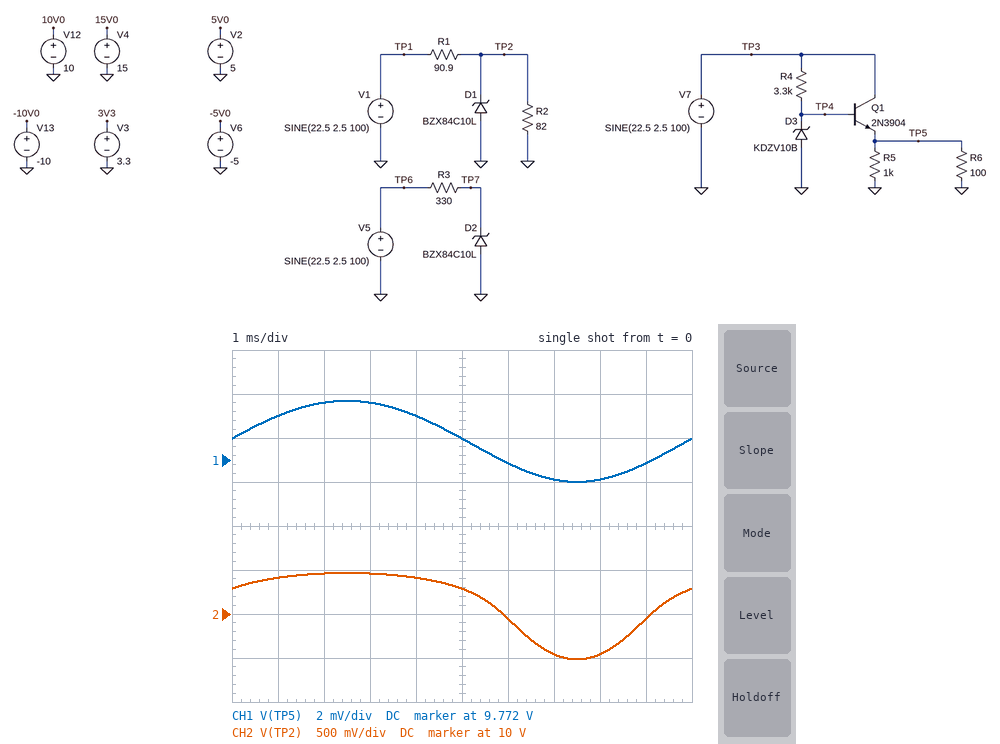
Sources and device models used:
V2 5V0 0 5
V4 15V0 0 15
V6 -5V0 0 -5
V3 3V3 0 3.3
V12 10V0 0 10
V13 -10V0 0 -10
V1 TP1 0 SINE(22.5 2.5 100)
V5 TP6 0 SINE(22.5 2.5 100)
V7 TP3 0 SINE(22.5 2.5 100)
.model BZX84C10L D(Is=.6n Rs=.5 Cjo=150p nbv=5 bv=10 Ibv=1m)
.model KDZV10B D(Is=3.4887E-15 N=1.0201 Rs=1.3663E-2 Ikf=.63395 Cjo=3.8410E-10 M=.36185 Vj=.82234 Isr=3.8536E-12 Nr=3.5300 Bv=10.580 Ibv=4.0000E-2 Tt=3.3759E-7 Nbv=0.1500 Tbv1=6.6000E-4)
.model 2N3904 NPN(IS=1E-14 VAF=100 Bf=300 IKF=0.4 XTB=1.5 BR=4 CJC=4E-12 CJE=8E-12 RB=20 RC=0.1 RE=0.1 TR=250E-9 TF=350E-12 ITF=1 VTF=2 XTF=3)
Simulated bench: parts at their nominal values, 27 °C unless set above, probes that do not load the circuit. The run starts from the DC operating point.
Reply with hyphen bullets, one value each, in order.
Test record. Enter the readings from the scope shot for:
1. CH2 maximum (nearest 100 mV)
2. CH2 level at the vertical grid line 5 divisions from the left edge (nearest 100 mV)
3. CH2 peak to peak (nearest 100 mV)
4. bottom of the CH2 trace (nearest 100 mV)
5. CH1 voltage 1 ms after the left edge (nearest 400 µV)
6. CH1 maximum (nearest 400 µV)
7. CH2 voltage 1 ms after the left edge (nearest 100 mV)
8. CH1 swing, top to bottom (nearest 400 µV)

- 10.5 V
- 10.3 V
- 1.0 V
- 9.5 V
- 9.7740 V
- 9.7748 V
- 10.4 V
- 3.6 mV
